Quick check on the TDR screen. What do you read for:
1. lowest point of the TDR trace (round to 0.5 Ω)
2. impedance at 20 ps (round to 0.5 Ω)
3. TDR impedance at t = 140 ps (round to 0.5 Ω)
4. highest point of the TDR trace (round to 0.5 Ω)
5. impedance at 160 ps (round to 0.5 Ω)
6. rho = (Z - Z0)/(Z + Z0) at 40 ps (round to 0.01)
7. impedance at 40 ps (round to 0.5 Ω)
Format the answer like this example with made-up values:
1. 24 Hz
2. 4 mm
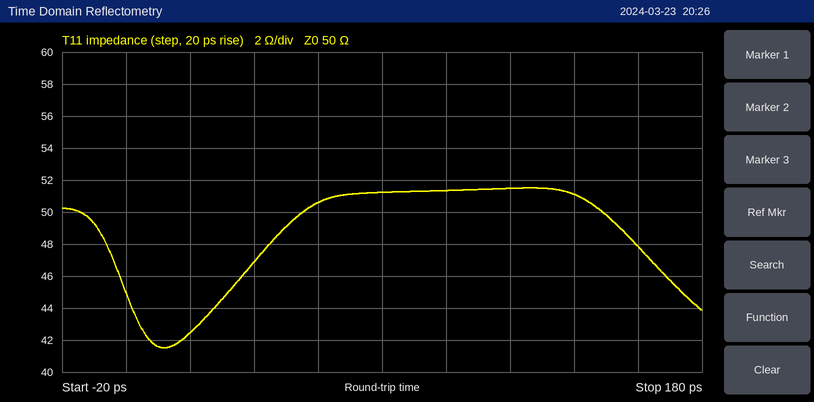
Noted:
1. 41.5 Ω
2. 42.5 Ω
3. 51.0 Ω
4. 51.5 Ω
5. 48.0 Ω
6. -0.03
7. 47.0 Ω
